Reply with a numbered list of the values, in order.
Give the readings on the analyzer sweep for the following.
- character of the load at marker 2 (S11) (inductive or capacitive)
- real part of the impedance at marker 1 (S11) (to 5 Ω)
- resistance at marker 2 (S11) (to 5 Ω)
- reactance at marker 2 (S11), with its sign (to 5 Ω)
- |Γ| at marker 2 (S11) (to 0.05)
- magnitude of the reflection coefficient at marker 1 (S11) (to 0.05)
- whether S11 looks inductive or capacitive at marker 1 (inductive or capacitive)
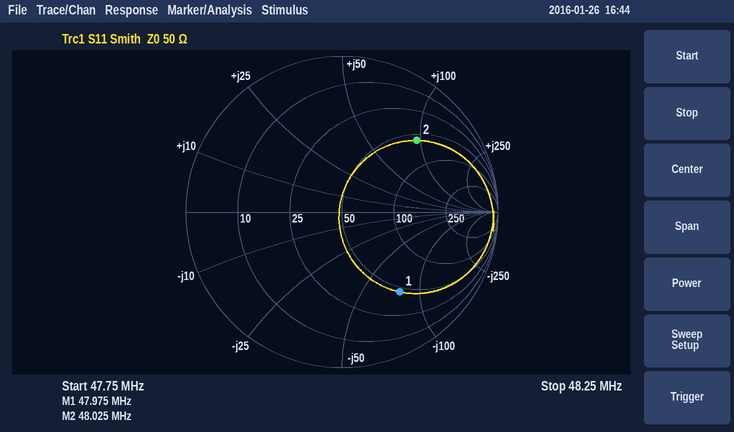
1. inductive
2. 45 Ω
3. 60 Ω
4. +95 Ω
5. 0.65
6. 0.65
7. capacitive
